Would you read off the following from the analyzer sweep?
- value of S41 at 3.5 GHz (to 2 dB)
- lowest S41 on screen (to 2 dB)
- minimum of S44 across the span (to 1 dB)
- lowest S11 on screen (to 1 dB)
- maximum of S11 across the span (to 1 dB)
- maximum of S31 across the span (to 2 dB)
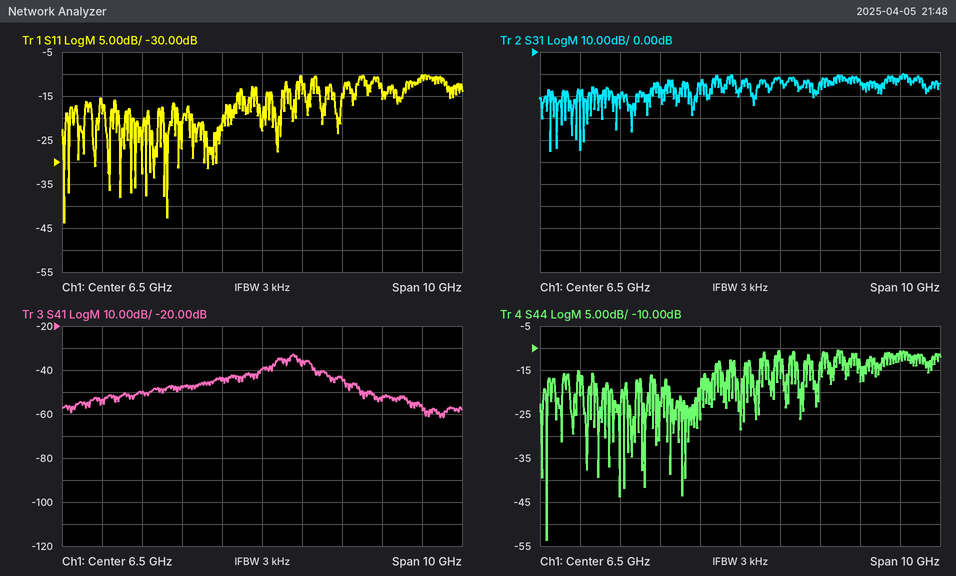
-50 dB
-62 dB
-54 dB
-44 dB
-10 dB
-10 dB
